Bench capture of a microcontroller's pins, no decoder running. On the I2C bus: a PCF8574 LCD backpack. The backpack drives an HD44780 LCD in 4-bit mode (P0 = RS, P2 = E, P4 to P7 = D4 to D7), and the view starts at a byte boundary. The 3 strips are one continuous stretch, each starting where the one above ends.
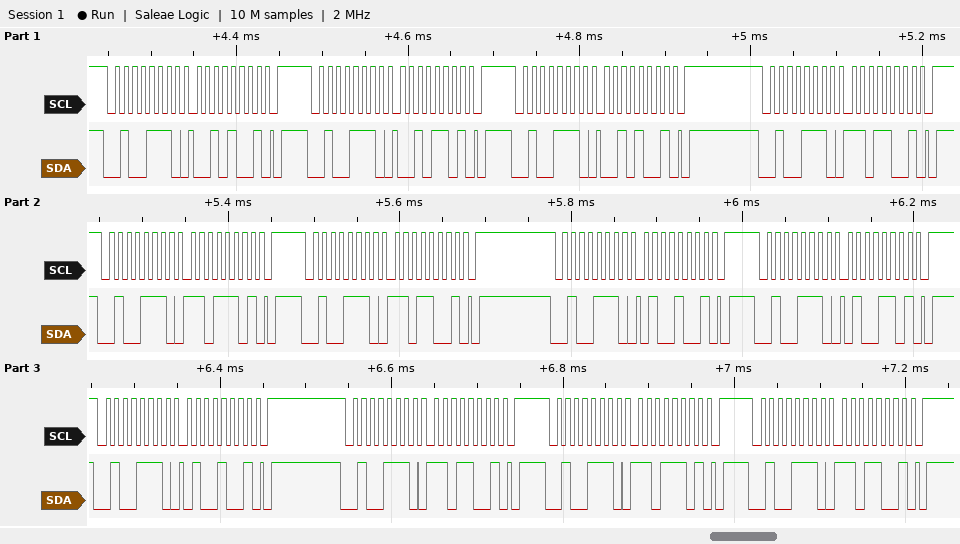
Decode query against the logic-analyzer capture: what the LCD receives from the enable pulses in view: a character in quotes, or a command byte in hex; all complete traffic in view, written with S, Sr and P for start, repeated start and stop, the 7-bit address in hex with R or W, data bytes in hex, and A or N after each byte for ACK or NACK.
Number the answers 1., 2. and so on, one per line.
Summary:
1. '-' 'M'
2. S 27W A 29 A P S 27W A 2D A P S 27W A 29 A P S 27W A D9 A P S 27W A DD A P S 27W A D9 A P S 27W A 49 A P S 27W A 4D A P S 27W A 49 A P S 27W A D9 A P S 27W A DD A P S 27W A D9 A P
